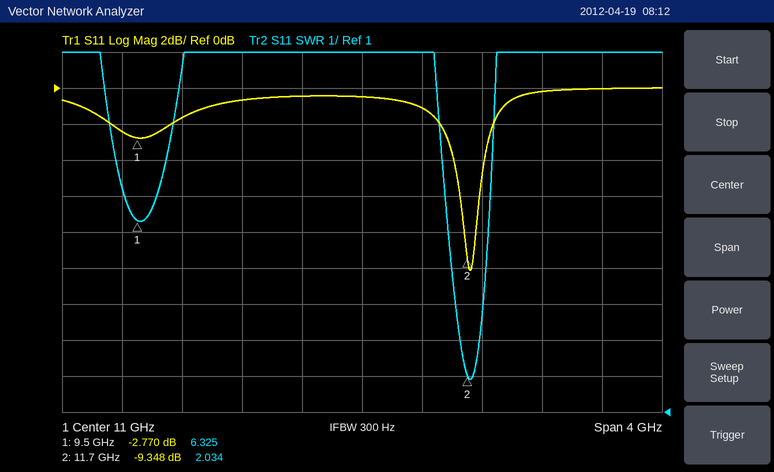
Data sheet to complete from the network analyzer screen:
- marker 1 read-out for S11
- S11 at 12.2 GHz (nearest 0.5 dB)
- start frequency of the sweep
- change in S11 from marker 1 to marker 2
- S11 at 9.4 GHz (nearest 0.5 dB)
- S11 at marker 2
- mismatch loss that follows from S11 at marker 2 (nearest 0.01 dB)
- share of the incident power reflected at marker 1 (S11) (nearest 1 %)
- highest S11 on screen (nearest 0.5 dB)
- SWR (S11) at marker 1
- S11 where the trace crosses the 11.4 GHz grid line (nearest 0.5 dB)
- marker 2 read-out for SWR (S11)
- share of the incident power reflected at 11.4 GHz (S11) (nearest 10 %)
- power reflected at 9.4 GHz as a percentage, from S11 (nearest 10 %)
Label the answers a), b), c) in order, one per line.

a) -2.770 dB
b) 0.0 dB
c) 9 GHz
d) -6.578 dB
e) -2.5 dB
f) -9.348 dB
g) 0.54 dB
h) 53 %
i) 0.0 dB
j) 6.325
k) -1.0 dB
l) 2.034
m) 80 %
n) 60 %
